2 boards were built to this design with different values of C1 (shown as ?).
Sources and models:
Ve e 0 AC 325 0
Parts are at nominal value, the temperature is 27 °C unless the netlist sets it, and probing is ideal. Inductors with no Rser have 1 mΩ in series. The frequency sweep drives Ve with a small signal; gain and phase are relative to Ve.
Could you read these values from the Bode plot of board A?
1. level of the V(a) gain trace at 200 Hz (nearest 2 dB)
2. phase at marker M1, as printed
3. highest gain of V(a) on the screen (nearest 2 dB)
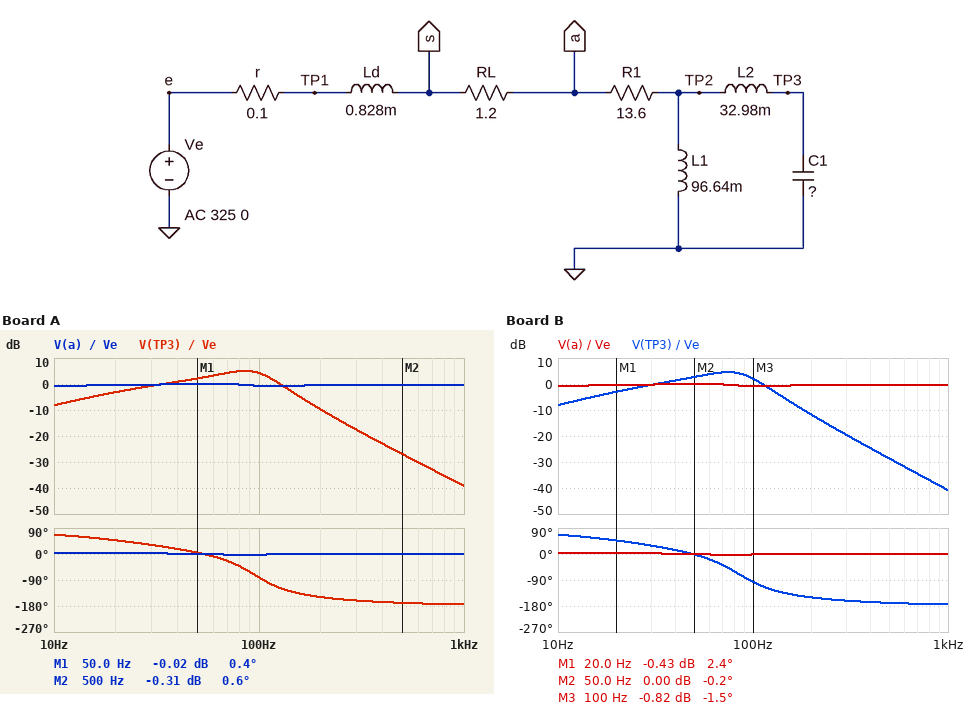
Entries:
0 dB
0.4 deg
0 dB
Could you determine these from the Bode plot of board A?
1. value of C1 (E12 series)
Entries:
68 µF
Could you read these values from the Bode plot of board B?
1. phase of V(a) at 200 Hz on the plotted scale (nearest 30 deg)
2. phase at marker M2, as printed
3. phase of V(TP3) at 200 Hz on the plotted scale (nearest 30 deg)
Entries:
0 deg
-0.2 deg
-150 deg
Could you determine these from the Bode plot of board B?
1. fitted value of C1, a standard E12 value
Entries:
82 µF
